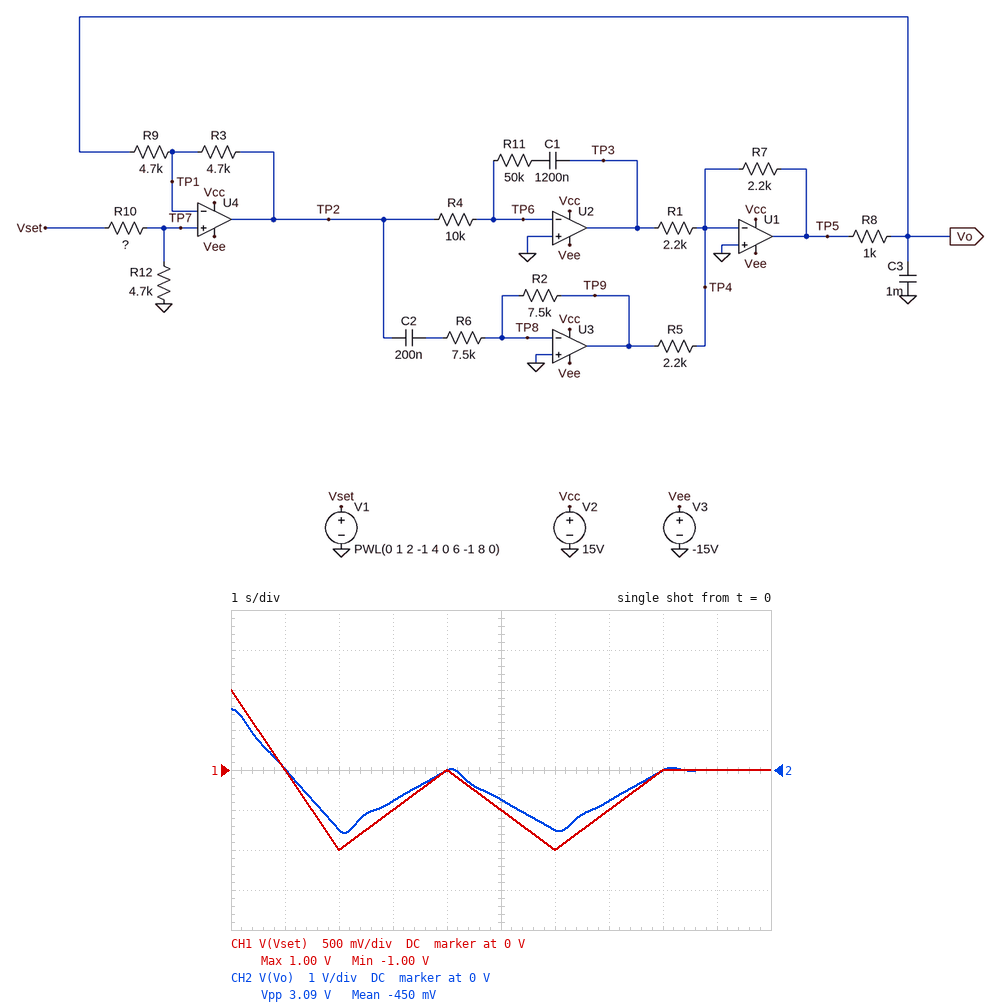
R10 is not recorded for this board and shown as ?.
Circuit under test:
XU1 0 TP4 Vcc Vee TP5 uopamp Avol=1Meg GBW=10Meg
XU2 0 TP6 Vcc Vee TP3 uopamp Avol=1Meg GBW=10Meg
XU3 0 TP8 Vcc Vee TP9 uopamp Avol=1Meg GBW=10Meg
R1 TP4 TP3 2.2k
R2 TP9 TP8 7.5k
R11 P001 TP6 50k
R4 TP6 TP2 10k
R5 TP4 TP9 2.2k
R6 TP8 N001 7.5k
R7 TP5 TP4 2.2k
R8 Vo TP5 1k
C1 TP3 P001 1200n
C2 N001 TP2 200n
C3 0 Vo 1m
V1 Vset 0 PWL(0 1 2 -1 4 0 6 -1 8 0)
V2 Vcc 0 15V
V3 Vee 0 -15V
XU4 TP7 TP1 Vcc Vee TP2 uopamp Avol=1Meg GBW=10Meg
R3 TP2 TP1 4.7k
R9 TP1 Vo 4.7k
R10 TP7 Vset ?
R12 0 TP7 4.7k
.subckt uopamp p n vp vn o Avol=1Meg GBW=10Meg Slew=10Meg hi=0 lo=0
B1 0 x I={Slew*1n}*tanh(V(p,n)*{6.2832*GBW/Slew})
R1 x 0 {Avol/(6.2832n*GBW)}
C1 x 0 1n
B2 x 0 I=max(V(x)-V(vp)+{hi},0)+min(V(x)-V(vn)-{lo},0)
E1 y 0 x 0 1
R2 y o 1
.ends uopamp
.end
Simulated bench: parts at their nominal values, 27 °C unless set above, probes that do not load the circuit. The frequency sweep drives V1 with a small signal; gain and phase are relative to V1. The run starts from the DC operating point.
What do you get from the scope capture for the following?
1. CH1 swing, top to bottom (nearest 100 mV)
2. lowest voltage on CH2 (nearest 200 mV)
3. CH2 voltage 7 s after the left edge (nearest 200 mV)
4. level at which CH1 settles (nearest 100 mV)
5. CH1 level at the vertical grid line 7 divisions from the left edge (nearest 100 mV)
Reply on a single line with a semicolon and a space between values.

2.0 V; -1.6 V; -800 mV; 0 V; -500 mV
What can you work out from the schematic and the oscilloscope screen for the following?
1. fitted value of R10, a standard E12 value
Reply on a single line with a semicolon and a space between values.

1.5 kΩ
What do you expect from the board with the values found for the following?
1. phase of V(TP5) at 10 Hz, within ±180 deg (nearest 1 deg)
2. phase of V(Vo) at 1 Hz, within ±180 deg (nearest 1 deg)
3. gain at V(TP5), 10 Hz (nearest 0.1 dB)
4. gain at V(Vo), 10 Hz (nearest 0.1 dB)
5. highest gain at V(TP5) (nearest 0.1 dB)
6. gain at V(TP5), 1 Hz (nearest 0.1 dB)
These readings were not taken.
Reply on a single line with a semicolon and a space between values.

-9 deg; -21 deg; 18.0 dB; -17.8 dB; 27.4 dB; 23.3 dB
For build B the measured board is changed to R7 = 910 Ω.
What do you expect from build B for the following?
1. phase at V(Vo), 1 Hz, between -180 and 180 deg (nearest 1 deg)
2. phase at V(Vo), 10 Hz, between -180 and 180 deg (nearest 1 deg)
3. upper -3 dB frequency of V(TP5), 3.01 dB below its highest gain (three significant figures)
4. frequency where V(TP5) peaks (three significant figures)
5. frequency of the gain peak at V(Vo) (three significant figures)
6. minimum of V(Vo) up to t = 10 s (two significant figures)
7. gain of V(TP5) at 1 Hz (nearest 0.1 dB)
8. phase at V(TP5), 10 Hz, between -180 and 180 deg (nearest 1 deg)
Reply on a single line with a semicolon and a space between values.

-82 deg; -100 deg; 1.25 Hz; 940 mHz; 867 mHz; -1.6 V; 24.5 dB; -12 deg
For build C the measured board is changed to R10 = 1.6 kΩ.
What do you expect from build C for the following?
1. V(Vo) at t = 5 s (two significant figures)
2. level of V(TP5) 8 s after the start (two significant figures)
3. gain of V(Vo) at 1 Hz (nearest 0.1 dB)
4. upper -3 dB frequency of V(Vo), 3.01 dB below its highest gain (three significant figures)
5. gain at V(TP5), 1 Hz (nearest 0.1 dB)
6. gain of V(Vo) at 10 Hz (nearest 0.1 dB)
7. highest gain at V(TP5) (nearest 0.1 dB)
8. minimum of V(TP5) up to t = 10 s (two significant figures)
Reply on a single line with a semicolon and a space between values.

-730 mV; 730 mV; 7.1 dB; 1.79 Hz; 23.2 dB; -17.9 dB; 27.2 dB; -3.1 V
